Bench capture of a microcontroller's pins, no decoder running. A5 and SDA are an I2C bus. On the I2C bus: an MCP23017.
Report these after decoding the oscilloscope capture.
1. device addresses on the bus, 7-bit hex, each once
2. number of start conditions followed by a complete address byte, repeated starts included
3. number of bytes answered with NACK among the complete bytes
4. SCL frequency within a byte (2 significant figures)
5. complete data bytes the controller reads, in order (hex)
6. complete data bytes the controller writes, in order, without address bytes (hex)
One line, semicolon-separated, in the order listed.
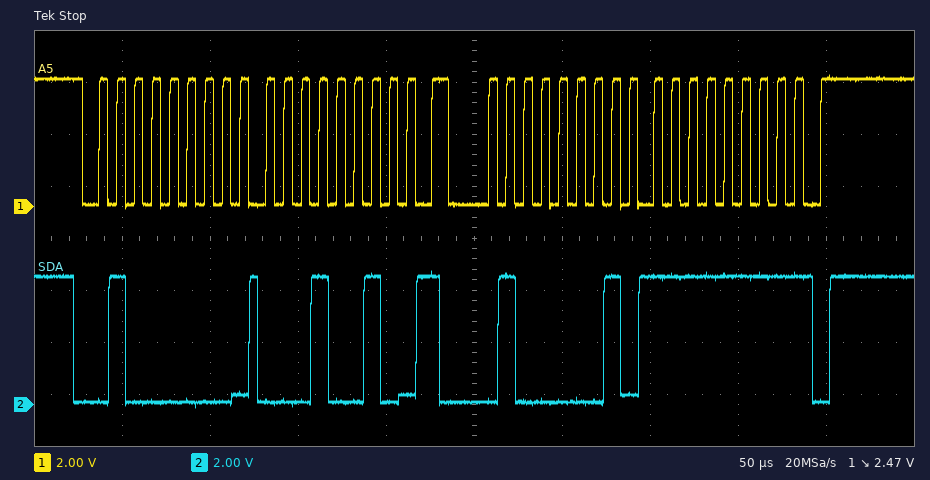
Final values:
0x20; 2; 1; 100 kHz; FF; 12
